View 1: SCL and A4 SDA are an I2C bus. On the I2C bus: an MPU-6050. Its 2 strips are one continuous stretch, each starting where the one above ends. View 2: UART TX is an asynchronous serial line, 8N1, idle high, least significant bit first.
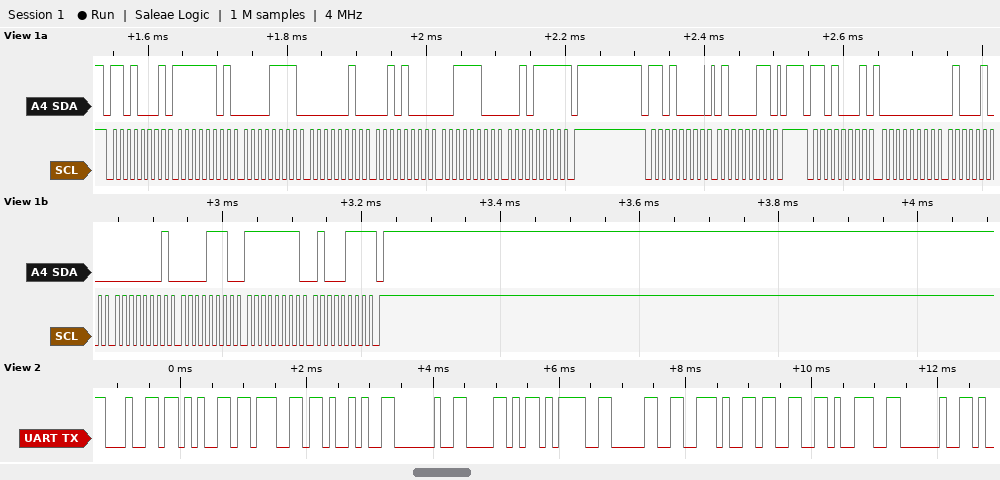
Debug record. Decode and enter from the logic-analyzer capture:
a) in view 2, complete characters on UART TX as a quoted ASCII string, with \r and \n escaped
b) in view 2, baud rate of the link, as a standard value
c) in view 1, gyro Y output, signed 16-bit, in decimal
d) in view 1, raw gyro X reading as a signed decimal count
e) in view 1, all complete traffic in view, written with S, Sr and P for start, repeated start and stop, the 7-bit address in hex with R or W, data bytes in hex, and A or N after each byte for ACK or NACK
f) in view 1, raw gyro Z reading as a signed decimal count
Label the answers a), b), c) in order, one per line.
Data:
a) "deg) X=0.39 "
b) 9600 baud
c) 270
d) 68
e) S 68R A FD A 0F A 02 A 28 A 3C A 2F N P S 68W A 43 A P S 68R A 00 A 44 A 01 A 0E A FF A 47 N P
f) -185
